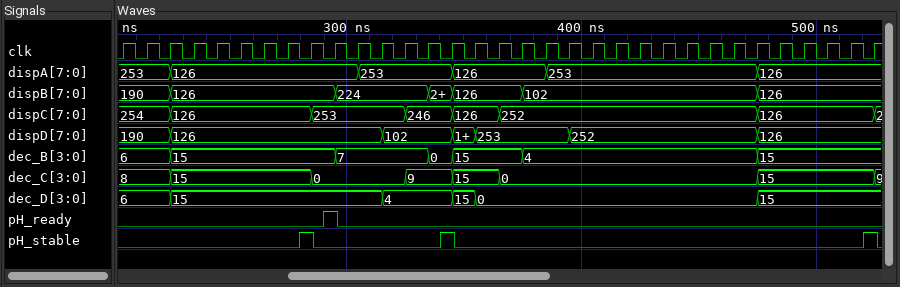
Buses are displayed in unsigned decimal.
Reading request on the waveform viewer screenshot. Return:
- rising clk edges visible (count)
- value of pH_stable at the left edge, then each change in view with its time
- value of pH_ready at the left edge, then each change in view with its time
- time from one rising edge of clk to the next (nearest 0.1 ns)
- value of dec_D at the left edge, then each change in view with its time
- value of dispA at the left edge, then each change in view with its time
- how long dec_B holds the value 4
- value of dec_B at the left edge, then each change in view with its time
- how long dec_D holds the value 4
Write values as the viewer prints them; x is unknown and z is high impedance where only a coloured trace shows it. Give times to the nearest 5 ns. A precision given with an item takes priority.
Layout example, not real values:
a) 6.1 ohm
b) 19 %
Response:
a) 33
b) 0, 1 at 280 ns, 0 at 285 ns, 1 at 340 ns, 0 at 345 ns, 1 at 520 ns, 0 at 525 ns
c) 0, 1 at 290 ns, 0 at 295 ns
d) 10 ns
e) 6, 15 at 225 ns, 4 at 315 ns, 15 at 345 ns, 0 at 355 ns, 15 at 475 ns
f) 253, 126 at 225 ns, 253 at 305 ns, 126 at 345 ns, 253 at 385 ns, 126 at 475 ns
g) 100 ns
h) 6, 15 at 225 ns, 7 at 295 ns, 0 at 335 ns, 15 at 345 ns, 4 at 375 ns, 15 at 475 ns
i) 30 ns
